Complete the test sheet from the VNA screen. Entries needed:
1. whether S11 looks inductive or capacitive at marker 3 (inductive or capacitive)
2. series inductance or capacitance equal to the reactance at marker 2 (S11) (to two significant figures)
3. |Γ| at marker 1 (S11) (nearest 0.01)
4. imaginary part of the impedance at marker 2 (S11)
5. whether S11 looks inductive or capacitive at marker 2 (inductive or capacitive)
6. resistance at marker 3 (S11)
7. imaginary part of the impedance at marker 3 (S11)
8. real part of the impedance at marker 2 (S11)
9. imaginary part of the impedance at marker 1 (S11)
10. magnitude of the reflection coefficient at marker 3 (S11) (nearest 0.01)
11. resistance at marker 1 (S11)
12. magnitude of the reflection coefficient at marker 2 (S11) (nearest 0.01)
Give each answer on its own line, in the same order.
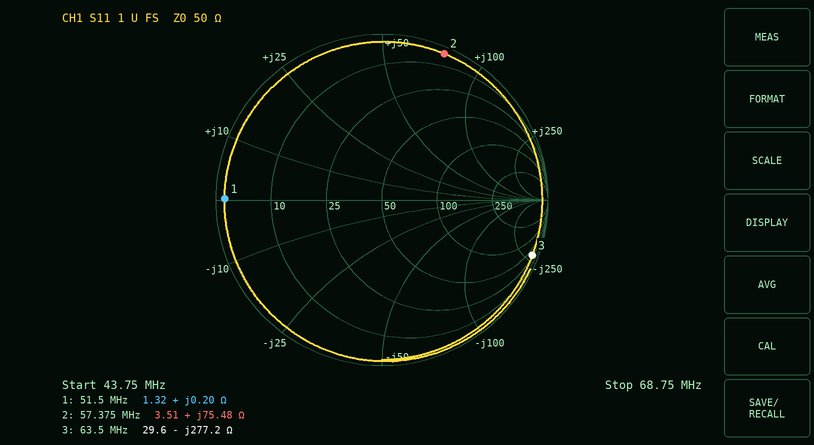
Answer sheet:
capacitive
210 nH
0.95
+75.48 Ω
inductive
29.6 Ω
-277.2 Ω
3.51 Ω
+0.20 Ω
0.96
1.32 Ω
0.96
